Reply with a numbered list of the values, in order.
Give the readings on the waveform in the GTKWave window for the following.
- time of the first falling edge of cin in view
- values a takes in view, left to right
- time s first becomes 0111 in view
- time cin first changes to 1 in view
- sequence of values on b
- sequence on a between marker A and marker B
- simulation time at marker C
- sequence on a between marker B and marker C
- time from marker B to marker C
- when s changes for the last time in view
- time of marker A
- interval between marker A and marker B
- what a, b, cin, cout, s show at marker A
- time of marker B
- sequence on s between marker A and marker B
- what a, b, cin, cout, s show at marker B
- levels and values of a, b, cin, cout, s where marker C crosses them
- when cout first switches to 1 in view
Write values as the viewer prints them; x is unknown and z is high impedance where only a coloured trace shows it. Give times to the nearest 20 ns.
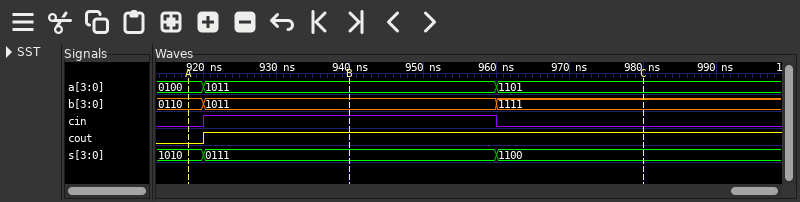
1. 960 ns
2. 0100, 1011, 1101
3. 920 ns
4. 920 ns
5. 0110, 1011, 1111
6. 0100, 1011
7. 980 ns
8. 1011, 1101
9. 40 ns
10. 960 ns
11. 920 ns
12. 20 ns
13. a=0100, b=0110, cin=0, cout=0, s=1010
14. 940 ns
15. 1010, 0111
16. a=1011, b=1011, cin=1, cout=1, s=0111
17. a=1101, b=1111, cin=0, cout=1, s=1100
18. 920 ns
